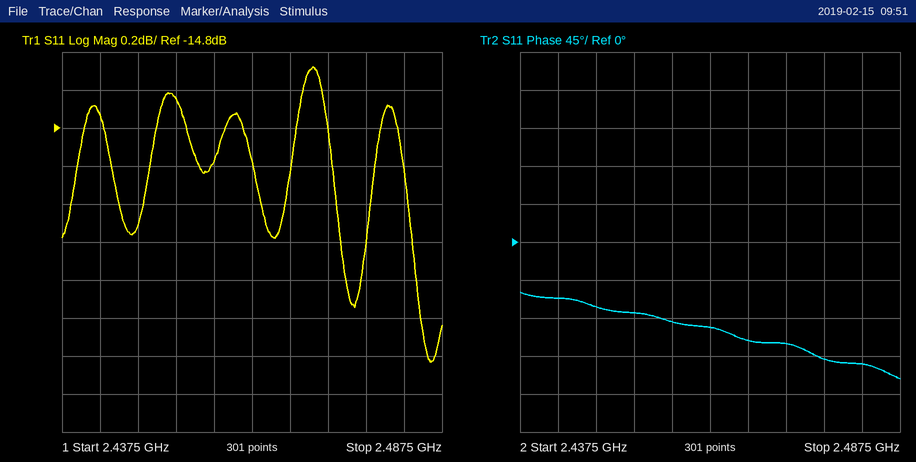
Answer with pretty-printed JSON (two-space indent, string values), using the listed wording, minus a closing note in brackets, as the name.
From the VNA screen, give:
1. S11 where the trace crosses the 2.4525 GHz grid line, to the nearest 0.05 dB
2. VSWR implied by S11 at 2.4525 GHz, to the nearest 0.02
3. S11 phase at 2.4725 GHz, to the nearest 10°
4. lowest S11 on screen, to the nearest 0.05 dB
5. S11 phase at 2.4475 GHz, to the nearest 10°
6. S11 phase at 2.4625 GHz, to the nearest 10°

{
  "S11 where the trace crosses the 2.4525 GHz grid line, to the nearest 0.05 dB": "-14.65 dB",
  "VSWR implied by S11 at 2.4525 GHz, to the nearest 0.02": "1.46",
  "S11 phase at 2.4725 GHz, to the nearest 10°": "-120°",
  "lowest S11 on screen, to the nearest 0.05 dB": "-16.05 dB",
  "S11 phase at 2.4475 GHz, to the nearest 10°": "-80°",
  "S11 phase at 2.4625 GHz, to the nearest 10°": "-100°"
}
